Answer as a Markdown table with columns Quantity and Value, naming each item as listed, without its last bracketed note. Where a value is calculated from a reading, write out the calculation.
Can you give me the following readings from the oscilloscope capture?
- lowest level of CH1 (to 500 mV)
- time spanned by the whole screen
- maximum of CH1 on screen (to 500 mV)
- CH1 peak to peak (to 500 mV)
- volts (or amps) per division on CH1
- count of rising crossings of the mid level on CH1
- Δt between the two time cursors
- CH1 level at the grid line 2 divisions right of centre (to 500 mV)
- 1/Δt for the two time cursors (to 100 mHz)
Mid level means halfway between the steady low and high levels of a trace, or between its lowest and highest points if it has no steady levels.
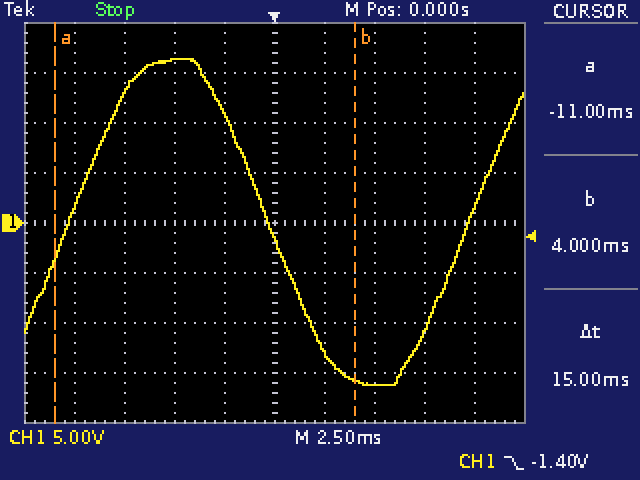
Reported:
| Quantity | Value |
|---|---|
| lowest level of CH1 | -16.0 V |
| time spanned by the whole screen | 25 ms |
| maximum of CH1 on screen | 16.5 V |
| CH1 peak to peak | 16.5 V − (-16.0 V) = 32.5 V |
| volts (or amps) per division on CH1 | 5 V |
| count of rising crossings of the mid level on CH1 | 2 |
| Δt between the two time cursors | 15 ms |
| CH1 level at the grid line 2 divisions right of centre | -16.0 V |
| 1/Δt for the two time cursors | 1 / 15 ms ≈ 66.7 Hz |
